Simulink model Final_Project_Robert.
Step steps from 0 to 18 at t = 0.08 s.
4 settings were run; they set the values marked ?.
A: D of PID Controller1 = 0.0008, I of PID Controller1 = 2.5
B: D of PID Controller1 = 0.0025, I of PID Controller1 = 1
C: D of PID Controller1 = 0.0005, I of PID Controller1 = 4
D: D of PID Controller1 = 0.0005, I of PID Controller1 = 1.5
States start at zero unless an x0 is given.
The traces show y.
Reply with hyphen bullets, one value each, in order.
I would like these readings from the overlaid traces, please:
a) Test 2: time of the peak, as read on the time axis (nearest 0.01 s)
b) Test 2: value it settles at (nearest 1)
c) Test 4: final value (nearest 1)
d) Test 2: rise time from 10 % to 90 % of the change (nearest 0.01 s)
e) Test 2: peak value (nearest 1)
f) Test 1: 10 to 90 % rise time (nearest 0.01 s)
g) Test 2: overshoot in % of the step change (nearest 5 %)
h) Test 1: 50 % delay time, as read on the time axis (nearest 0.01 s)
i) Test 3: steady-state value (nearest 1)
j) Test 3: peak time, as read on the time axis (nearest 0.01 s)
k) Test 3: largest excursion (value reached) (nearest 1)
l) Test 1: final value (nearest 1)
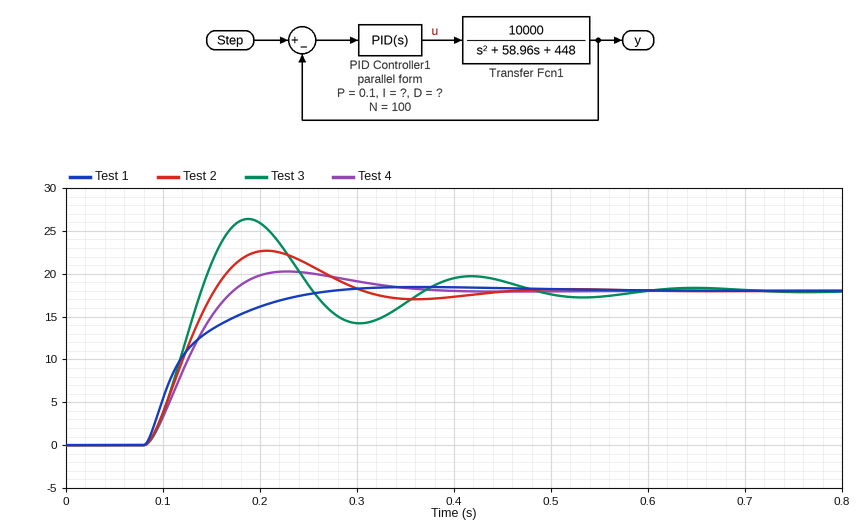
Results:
- 0.21 s
- 18
- 18
- 0.05 s
- 23
- 0.11 s
- 25 %
- 0.11 s
- 18
- 0.19 s
- 26
- 18
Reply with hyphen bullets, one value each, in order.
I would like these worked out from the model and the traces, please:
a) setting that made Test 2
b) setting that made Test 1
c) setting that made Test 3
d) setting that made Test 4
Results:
- A
- B
- C
- D
